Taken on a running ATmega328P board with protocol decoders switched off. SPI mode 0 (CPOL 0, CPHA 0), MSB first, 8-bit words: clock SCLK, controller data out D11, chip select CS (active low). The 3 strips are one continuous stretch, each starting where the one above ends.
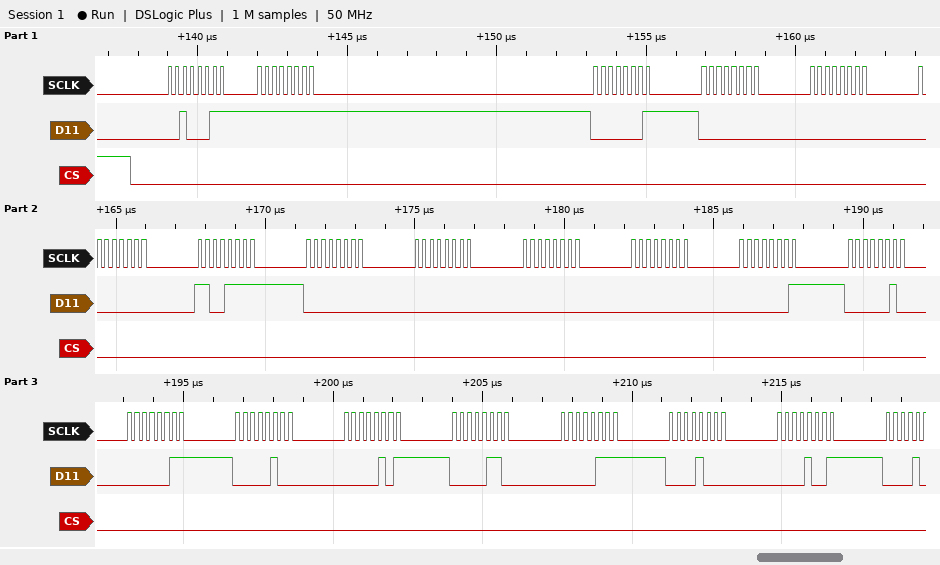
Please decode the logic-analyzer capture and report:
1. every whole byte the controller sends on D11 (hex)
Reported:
23 FF 01 00 00 00 CF 00 00 00 00 01 02 03 04 05 06 07 08 09
